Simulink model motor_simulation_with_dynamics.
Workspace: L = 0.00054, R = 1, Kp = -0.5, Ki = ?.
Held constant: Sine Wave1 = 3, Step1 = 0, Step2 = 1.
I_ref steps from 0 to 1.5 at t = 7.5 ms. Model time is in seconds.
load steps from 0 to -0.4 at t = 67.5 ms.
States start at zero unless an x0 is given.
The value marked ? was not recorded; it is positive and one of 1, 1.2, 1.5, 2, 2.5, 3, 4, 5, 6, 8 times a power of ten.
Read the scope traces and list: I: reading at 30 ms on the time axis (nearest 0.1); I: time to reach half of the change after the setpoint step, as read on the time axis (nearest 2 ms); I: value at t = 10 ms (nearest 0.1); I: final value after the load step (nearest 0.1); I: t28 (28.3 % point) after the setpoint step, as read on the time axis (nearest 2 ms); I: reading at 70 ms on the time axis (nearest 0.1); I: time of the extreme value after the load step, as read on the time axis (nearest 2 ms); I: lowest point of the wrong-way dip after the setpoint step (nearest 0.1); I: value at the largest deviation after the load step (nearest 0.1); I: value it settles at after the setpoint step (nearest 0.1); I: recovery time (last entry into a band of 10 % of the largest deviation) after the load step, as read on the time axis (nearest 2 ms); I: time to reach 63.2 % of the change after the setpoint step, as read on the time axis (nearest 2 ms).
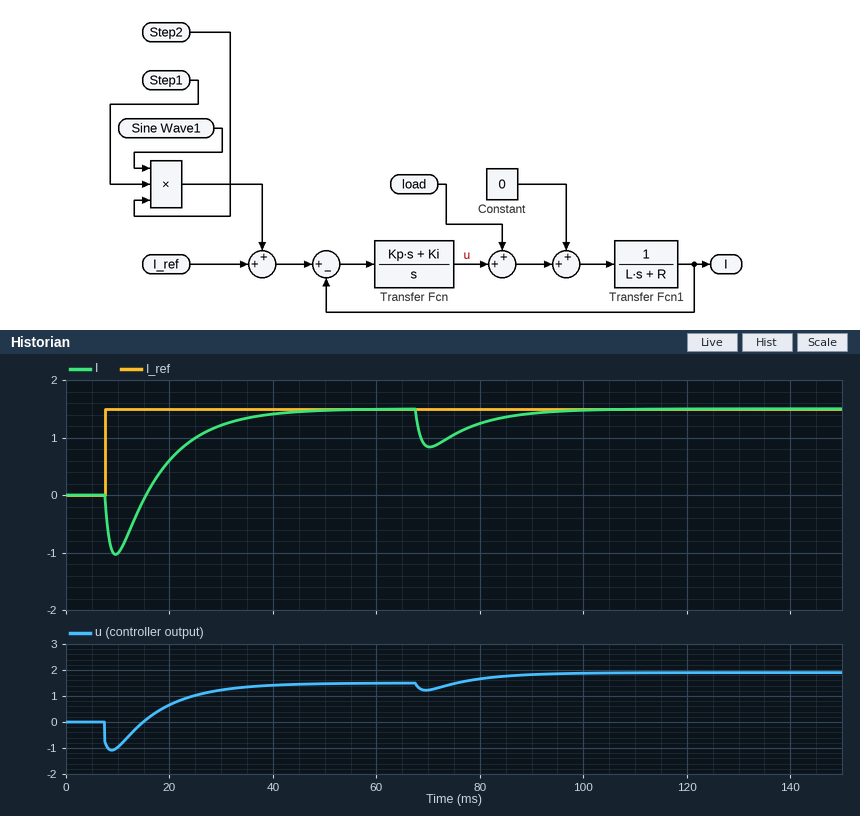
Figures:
1.2
22 ms
-1.0
1.5
18 ms
0.8
70 ms
-1.0
0.8
1.5
92 ms
24 ms
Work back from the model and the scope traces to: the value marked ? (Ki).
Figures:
50
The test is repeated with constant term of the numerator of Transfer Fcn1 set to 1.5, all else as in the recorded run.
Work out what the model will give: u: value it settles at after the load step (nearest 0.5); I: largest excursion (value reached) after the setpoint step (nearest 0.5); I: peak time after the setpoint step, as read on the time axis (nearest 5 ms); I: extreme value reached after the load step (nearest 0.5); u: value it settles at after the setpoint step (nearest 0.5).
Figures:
1.5
2.0
20 ms
0.0
1.0
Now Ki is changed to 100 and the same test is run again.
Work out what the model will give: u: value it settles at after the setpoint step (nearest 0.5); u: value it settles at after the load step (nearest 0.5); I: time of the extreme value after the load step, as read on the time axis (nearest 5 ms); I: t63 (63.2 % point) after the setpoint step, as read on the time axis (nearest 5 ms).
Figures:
1.5
2.0
70 ms
15 ms
